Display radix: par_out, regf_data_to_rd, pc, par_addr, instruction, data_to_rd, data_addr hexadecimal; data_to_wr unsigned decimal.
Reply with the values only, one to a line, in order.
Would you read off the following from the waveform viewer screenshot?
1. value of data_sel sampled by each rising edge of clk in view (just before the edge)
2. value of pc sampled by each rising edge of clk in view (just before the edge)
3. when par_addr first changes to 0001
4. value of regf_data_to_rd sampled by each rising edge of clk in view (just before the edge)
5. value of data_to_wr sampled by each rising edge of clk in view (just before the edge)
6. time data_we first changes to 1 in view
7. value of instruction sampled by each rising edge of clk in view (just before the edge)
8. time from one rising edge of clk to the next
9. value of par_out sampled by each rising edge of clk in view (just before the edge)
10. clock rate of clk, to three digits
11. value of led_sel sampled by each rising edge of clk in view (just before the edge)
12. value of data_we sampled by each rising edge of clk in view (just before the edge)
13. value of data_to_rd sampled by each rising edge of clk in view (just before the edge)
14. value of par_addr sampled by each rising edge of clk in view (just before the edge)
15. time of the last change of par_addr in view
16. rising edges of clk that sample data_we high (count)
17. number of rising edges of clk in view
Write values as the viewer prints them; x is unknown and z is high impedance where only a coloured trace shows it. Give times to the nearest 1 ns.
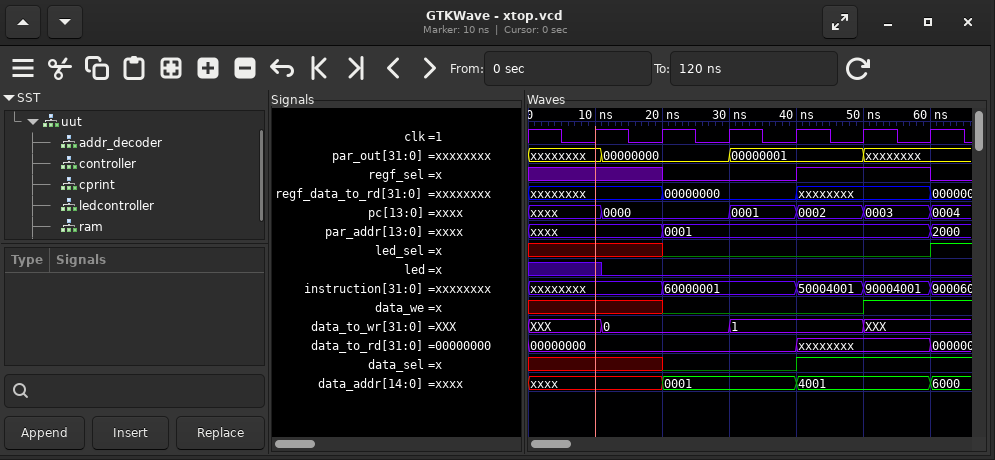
x x 0 0 1 1
xxxx, 0000, 0000, 0001, 0002, 0003
20 ns
xxxxxxxx, xxxxxxxx, 00000000, 00000000, xxxxxxxx, xxxxxxxx
XXX, 0, 0, 1, 1, XXX
50 ns
xxxxxxxx, xxxxxxxx, 60000001, 60000001, 50004001, 90004001
10 ns
xxxxxxxx, 00000000, 00000000, 00000001, 00000001, xxxxxxxx
100 MHz
x x 0 0 0 0
x x 0 0 0 1
00000000, 00000000, 00000000, 00000000, xxxxxxxx, xxxxxxxx
xxxx, xxxx, 0001, 0001, 0001, 0001
60 ns
1
6
